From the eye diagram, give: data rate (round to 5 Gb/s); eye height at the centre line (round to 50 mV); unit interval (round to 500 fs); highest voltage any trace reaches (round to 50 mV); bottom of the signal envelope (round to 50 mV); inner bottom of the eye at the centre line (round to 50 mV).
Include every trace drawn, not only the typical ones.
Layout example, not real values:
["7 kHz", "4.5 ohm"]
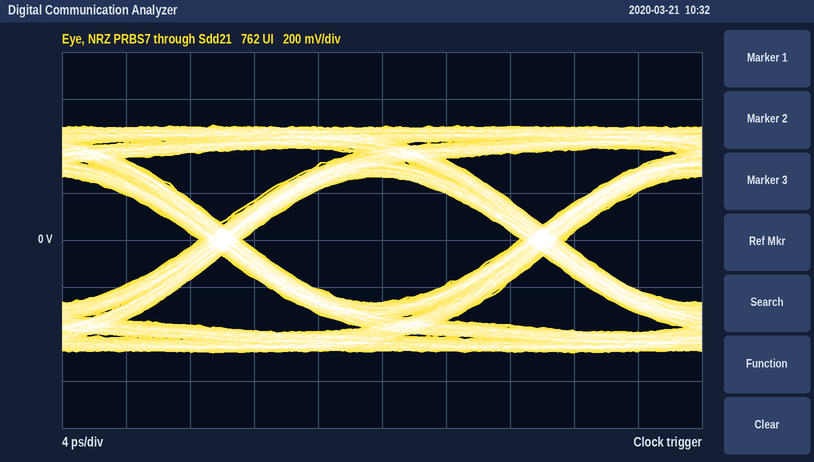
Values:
["50 Gb/s", "550 mV", "20.0 ps", "500 mV", "-500 mV", "-250 mV"]
